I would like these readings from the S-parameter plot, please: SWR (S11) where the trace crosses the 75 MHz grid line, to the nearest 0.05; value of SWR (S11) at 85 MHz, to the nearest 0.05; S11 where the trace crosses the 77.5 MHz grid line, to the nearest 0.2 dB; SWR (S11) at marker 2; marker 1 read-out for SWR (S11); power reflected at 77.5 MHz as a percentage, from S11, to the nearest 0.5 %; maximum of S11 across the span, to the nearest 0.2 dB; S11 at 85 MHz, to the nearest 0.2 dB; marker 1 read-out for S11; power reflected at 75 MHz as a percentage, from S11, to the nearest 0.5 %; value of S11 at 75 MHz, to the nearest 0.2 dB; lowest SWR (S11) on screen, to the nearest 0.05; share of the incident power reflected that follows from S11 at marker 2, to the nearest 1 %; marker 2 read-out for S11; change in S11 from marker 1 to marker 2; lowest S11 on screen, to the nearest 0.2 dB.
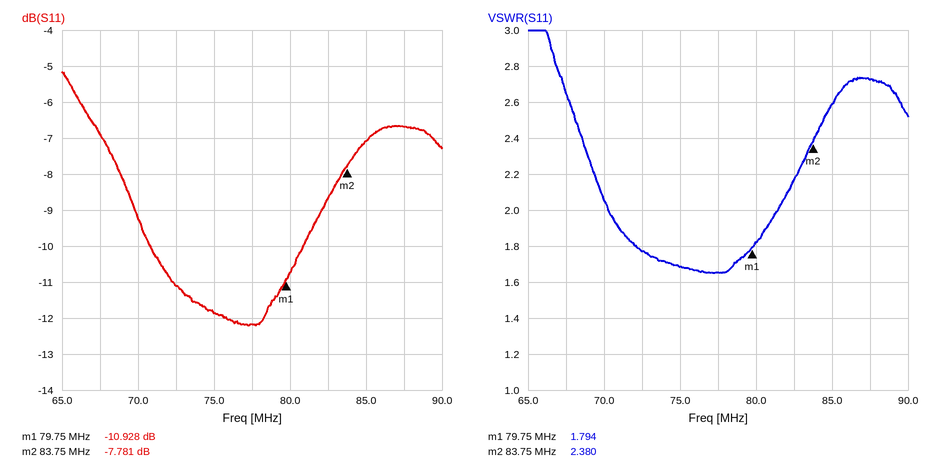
1.70
2.60
-12.2 dB
2.380
1.794
6.0 %
-5.2 dB
-7.0 dB
-10.928 dB
6.5 %
-11.8 dB
1.65
17 %
-7.781 dB
3.147 dB
-12.2 dB
